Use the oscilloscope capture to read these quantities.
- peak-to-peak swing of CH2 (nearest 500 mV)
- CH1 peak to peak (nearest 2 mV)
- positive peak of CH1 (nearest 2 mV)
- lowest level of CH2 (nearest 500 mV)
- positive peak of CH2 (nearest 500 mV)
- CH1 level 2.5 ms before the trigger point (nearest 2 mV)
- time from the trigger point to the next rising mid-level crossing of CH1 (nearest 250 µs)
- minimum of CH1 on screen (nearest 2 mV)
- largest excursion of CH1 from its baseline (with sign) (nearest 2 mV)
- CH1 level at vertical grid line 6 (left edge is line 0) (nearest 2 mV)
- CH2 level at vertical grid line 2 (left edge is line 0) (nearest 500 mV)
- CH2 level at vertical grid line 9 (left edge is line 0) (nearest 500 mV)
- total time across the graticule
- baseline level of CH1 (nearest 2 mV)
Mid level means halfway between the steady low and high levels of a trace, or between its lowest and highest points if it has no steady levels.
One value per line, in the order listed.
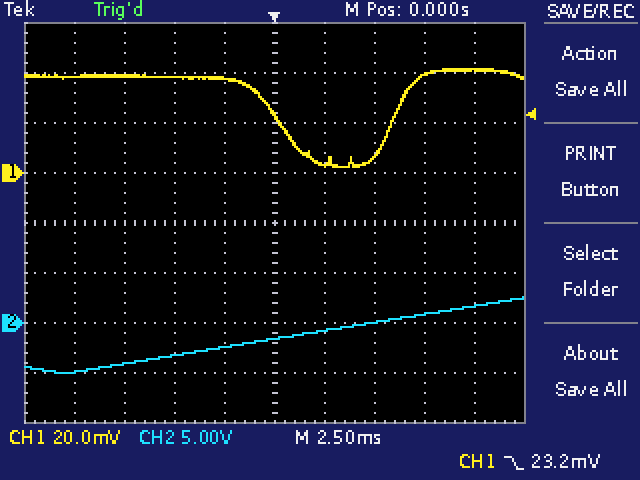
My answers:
7.5 V
40 mV
42 mV
-5.0 V
2.5 V
38 mV
6.00 ms
2 mV
-36 mV
4 mV
-4.0 V
1.5 V
25 ms
38 mV
